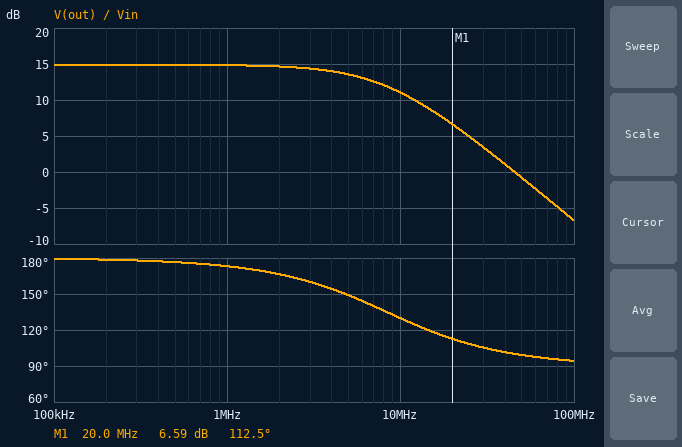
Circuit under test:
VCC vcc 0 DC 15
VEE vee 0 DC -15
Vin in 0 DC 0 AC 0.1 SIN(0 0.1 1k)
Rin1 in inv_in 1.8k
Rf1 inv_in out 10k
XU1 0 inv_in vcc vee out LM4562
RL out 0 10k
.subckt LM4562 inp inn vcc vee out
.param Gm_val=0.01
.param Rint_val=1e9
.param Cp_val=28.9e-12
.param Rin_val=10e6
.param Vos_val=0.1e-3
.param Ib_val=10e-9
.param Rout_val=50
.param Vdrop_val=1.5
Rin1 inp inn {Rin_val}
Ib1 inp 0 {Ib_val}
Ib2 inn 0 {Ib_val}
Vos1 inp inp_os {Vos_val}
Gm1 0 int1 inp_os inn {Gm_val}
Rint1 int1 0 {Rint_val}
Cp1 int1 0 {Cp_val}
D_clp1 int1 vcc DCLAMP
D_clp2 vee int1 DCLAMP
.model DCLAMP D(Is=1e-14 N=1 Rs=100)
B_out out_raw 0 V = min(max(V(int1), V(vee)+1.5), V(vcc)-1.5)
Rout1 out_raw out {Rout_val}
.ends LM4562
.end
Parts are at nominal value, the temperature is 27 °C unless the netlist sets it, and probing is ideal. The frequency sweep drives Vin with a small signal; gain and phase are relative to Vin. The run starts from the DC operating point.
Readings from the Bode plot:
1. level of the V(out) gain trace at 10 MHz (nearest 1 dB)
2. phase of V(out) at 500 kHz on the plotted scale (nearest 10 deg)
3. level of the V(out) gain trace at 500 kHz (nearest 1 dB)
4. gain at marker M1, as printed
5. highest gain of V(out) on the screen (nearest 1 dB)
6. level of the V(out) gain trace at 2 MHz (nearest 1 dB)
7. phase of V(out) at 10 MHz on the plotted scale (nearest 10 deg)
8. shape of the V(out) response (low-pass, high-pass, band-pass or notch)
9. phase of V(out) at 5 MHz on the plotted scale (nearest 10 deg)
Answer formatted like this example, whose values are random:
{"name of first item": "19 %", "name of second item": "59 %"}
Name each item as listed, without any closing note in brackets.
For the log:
{"level of the V(out) gain trace at 10 MHz": "11 dB", "phase of V(out) at 500 kHz on the plotted scale": "180 deg", "level of the V(out) gain trace at 500 kHz": "15 dB", "gain at marker M1, as printed": "6.59 dB", "highest gain of V(out) on the screen": "15 dB", "level of the V(out) gain trace at 2 MHz": "15 dB", "phase of V(out) at 10 MHz on the plotted scale": "130 deg", "shape of the V(out) response": "low-pass", "phase of V(out) at 5 MHz on the plotted scale": "150 deg"}
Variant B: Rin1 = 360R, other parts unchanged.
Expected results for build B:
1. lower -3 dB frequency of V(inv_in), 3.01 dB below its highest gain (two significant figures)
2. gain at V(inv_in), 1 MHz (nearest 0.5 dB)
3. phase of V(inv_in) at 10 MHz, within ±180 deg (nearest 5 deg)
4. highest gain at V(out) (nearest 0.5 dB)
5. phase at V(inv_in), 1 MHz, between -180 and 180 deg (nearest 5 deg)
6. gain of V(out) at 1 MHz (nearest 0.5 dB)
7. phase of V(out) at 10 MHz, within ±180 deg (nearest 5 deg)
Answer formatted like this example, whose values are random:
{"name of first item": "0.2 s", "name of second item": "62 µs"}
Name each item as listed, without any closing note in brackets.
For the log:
{"lower -3 dB frequency of V(inv_in), 3.01 dB below its highest gain": "1.9 MHz", "gain at V(inv_in), 1 MHz": "-7.0 dB", "phase of V(inv_in) at 10 MHz, within ±180 deg": "10 deg", "highest gain at V(out)": "29.0 dB", "phase at V(inv_in), 1 MHz, between -180 and 180 deg": "60 deg", "gain of V(out) at 1 MHz": "28.0 dB", "phase of V(out) at 10 MHz, within ±180 deg": "100 deg"}
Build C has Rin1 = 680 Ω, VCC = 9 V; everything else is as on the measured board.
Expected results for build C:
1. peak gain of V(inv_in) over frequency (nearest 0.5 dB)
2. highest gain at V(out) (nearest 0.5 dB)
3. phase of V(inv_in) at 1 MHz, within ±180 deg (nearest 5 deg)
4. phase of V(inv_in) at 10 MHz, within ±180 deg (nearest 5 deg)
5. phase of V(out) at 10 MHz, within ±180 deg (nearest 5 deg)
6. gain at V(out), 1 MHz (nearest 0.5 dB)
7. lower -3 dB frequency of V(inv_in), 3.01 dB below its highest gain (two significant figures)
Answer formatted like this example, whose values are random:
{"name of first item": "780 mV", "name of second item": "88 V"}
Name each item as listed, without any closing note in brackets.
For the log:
{"peak gain of V(inv_in) over frequency": "-0.5 dB", "highest gain at V(out)": "23.5 dB", "phase of V(inv_in) at 1 MHz, within ±180 deg": "75 deg", "phase of V(inv_in) at 10 MHz, within ±180 deg": "20 deg", "phase of V(out) at 10 MHz, within ±180 deg": "110 deg", "gain at V(out), 1 MHz": "23.0 dB", "lower -3 dB frequency of V(inv_in), 3.01 dB below its highest gain": "3.5 MHz"}
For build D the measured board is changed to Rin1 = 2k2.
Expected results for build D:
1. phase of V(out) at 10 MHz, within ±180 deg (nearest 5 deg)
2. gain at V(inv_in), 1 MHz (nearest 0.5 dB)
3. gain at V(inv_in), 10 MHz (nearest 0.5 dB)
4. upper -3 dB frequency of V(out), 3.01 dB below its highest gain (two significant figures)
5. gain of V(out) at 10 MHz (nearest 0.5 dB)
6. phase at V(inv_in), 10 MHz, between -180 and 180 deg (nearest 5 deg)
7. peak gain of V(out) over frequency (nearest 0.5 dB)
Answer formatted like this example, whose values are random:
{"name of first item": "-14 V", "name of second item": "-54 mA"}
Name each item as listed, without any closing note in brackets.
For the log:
{"phase of V(out) at 10 MHz, within ±180 deg": "135 deg", "gain at V(inv_in), 1 MHz": "-21.5 dB", "gain at V(inv_in), 10 MHz": "-4.5 dB", "upper -3 dB frequency of V(out), 3.01 dB below its highest gain": "9.8 MHz", "gain of V(out) at 10 MHz": "10.0 dB", "phase at V(inv_in), 10 MHz, between -180 and 180 deg": "45 deg", "peak gain of V(out) over frequency": "13.0 dB"}
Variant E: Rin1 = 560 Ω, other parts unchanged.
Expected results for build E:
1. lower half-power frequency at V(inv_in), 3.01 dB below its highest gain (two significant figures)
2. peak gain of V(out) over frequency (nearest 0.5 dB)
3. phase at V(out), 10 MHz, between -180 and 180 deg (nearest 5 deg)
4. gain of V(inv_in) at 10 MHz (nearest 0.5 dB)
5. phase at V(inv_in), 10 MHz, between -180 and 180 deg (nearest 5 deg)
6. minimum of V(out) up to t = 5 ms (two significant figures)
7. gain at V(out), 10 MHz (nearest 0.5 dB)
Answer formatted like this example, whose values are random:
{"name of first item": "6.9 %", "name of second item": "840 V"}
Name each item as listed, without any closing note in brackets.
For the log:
{"lower half-power frequency at V(inv_in), 3.01 dB below its highest gain": "2.9 MHz", "peak gain of V(out) over frequency": "25.0 dB", "phase at V(out), 10 MHz, between -180 and 180 deg": "105 deg", "gain of V(inv_in) at 10 MHz": "-1.0 dB", "phase at V(inv_in), 10 MHz, between -180 and 180 deg": "15 deg", "minimum of V(out) up to t = 5 ms": "-1.8 V", "gain at V(out), 10 MHz": "14.0 dB"}
